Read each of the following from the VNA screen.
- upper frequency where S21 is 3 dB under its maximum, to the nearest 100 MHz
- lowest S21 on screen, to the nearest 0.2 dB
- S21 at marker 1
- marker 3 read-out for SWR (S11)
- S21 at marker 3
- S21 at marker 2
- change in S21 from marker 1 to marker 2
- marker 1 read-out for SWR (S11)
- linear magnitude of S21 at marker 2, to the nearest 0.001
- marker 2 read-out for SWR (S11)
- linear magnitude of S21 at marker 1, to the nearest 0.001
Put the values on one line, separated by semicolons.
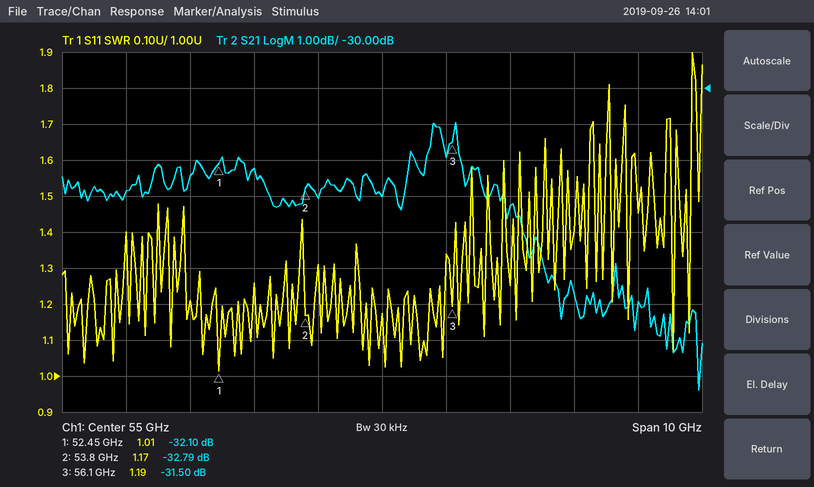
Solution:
57.2 GHz; -38.4 dB; -32.10 dB; 1.19; -31.50 dB; -32.79 dB; -0.69 dB; 1.01; 0.023; 1.17; 0.025
